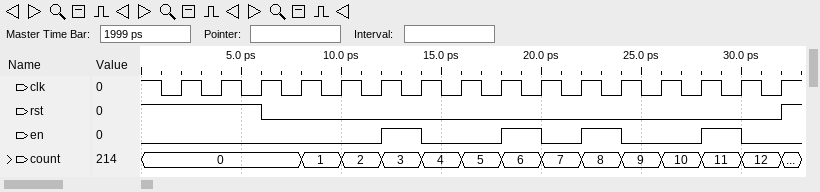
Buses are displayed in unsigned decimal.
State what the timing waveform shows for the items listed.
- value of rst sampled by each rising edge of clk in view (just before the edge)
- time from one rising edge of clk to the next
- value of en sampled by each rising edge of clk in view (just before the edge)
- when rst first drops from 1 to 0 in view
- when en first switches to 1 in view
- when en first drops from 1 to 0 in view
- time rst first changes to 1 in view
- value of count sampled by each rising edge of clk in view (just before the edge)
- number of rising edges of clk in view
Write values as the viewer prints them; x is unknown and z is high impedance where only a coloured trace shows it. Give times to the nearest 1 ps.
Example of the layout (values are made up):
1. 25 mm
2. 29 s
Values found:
1. 1 1 1 0 0 0 0 0 0 0 0 0 0 0 0 0
2. 2 ps
3. 0 0 0 0 0 0 1 0 0 1 0 1 0 0 1 0
4. 6 ps
5. 12 ps
6. 14 ps
7. 32 ps
8. 0, 0, 0, 0, 1, 2, 3, 4, 5, 6, 7, 8, 9, 10, 11, 12
9. 16
